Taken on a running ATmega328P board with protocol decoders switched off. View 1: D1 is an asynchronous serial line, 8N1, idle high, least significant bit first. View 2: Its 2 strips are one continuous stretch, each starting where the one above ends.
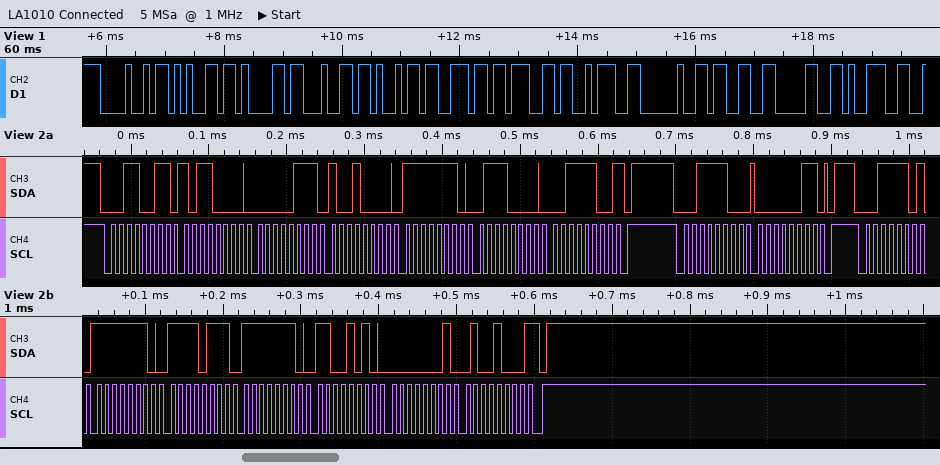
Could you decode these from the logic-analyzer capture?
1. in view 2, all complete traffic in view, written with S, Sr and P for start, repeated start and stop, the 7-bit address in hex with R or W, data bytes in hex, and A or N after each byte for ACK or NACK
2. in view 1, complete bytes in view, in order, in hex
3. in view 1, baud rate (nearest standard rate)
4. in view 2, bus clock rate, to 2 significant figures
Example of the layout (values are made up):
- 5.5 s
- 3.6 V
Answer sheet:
- S 19R A B0 A 07 A 90 A FE A 70 A 3C N P S 1EW A 03 A P S 1ER A FE A F7 A FE A CA A 01 A 48 N P
- 48 65 61 64 69 6E 67 3A 20 33 30 39
- 9600 baud
- 100 kHz
